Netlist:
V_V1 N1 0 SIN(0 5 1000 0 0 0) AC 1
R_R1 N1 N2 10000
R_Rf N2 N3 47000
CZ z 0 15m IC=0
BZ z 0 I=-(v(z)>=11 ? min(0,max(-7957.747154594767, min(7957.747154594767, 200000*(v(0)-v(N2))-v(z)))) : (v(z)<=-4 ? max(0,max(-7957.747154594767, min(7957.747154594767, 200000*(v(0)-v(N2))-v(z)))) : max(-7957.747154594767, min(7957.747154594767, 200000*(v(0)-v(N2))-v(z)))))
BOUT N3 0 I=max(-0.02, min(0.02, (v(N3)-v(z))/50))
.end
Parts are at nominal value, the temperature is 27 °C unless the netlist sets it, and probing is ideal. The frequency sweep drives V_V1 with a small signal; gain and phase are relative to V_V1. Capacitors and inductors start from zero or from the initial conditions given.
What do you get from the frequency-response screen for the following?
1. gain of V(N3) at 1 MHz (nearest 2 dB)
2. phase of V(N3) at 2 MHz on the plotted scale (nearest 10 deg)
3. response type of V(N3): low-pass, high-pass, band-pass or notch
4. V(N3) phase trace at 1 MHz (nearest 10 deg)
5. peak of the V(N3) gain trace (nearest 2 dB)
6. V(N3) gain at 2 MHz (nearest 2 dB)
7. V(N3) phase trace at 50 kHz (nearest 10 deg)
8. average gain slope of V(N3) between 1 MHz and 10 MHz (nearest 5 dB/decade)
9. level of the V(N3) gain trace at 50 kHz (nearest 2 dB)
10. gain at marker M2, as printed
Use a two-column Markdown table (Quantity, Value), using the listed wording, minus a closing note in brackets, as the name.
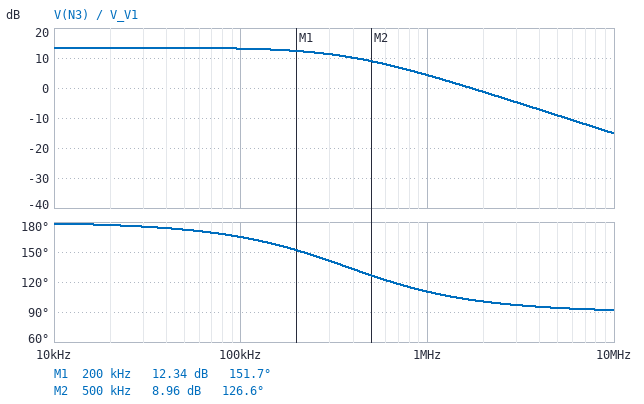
| Quantity | Value |
|---|---|
| gain of V(N3) at 1 MHz | 4 dB |
| phase of V(N3) at 2 MHz on the plotted scale | 100 deg |
| response type of V(N3): low-pass, high-pass, band-pass or notch | low-pass |
| V(N3) phase trace at 1 MHz | 110 deg |
| peak of the V(N3) gain trace | 14 dB |
| V(N3) gain at 2 MHz | -2 dB |
| V(N3) phase trace at 50 kHz | 170 deg |
| average gain slope of V(N3) between 1 MHz and 10 MHz | -20 dB/decade |
| level of the V(N3) gain trace at 50 kHz | 14 dB |
| gain at marker M2, as printed | 8.96 dB |
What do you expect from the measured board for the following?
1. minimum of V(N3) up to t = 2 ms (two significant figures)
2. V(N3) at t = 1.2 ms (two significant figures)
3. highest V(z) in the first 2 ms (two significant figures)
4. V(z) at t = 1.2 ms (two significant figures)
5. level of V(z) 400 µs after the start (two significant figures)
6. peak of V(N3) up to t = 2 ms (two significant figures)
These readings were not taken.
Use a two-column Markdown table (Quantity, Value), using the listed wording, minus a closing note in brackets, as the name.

| Quantity | Value |
|---|---|
| minimum of V(N3) up to t = 2 ms | -4.0 V |
| V(N3) at t = 1.2 ms | -4.0 V |
| highest V(z) in the first 2 ms | 11 V |
| V(z) at t = 1.2 ms | -4.0 V |
| level of V(z) 400 µs after the start | -4.0 V |
| peak of V(N3) up to t = 2 ms | 11 V |
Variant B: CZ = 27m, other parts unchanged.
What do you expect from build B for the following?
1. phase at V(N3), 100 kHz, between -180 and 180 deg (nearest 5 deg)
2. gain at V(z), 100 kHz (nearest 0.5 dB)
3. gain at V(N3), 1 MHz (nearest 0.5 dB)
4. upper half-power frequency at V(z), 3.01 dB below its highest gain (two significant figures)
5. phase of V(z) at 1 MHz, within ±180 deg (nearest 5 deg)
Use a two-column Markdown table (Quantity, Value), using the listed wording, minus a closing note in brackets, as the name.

| Quantity | Value |
|---|---|
| phase at V(N3), 100 kHz, between -180 and 180 deg | 155 deg |
| gain at V(z), 100 kHz | 12.5 dB |
| gain at V(N3), 1 MHz | -0.5 dB |
| upper half-power frequency at V(z), 3.01 dB below its highest gain | 210 kHz |
| phase of V(z) at 1 MHz, within ±180 deg | 100 deg |
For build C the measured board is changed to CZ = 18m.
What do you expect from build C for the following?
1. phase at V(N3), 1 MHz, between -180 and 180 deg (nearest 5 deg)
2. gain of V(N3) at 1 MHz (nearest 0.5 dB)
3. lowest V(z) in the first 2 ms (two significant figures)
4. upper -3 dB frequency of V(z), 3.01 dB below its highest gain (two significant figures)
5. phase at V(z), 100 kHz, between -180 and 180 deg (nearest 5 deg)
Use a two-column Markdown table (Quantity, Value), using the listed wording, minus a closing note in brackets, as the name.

| Quantity | Value |
|---|---|
| phase at V(N3), 1 MHz, between -180 and 180 deg | 105 deg |
| gain of V(N3) at 1 MHz | 3.0 dB |
| lowest V(z) in the first 2 ms | -4.0 V |
| upper -3 dB frequency of V(z), 3.01 dB below its highest gain | 310 kHz |
| phase at V(z), 100 kHz, between -180 and 180 deg | 160 deg |
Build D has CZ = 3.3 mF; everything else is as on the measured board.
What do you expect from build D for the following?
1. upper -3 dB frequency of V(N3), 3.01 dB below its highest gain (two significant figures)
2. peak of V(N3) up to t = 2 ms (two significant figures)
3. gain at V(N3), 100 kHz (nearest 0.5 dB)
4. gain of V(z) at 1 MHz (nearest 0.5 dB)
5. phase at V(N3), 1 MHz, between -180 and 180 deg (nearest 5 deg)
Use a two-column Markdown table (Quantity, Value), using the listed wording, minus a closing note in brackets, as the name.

| Quantity | Value |
|---|---|
| upper -3 dB frequency of V(N3), 3.01 dB below its highest gain | 1.7 MHz |
| peak of V(N3) up to t = 2 ms | 11 V |
| gain at V(N3), 100 kHz | 13.5 dB |
| gain of V(z) at 1 MHz | 12.0 dB |
| phase at V(N3), 1 MHz, between -180 and 180 deg | 150 deg |
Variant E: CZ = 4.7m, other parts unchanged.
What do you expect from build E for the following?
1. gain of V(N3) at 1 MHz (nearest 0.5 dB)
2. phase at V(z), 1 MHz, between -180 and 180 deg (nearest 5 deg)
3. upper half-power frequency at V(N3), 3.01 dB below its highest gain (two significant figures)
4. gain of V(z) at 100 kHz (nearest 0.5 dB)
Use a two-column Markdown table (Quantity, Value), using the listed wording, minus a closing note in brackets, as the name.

| Quantity | Value |
|---|---|
| gain of V(N3) at 1 MHz | 11.0 dB |
| phase at V(z), 1 MHz, between -180 and 180 deg | 140 deg |
| upper half-power frequency at V(N3), 3.01 dB below its highest gain | 1.2 MHz |
| gain of V(z) at 100 kHz | 13.5 dB |
